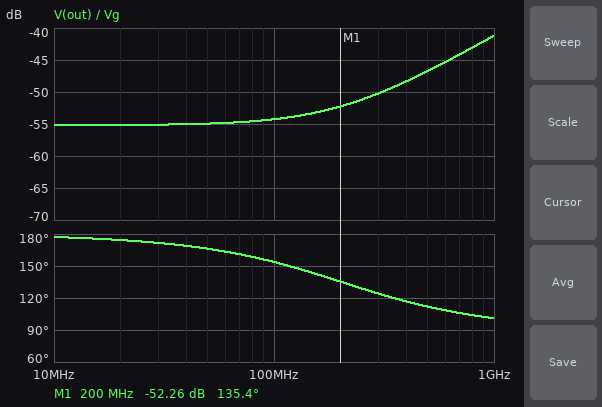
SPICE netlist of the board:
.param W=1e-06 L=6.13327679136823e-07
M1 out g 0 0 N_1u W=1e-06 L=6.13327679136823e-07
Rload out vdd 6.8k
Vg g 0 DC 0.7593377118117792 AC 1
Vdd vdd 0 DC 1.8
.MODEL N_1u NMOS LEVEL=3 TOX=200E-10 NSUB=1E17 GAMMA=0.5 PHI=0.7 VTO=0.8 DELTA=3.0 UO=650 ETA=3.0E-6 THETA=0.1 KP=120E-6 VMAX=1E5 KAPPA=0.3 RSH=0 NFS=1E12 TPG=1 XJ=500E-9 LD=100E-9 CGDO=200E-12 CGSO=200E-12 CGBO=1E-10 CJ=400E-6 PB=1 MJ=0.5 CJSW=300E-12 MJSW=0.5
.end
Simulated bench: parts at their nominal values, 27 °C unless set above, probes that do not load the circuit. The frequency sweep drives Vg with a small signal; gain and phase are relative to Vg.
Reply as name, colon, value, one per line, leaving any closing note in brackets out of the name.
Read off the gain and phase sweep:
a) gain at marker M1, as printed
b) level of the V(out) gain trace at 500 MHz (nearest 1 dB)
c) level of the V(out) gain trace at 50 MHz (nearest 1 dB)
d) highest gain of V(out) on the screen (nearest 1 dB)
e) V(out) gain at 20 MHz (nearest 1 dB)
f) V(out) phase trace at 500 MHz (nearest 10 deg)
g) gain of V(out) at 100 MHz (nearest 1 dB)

gain at marker M1, as printed: -52.26 dB
level of the V(out) gain trace at 500 MHz: -47 dB
level of the V(out) gain trace at 50 MHz: -55 dB
highest gain of V(out) on the screen: -41 dB
V(out) gain at 20 MHz: -55 dB
V(out) phase trace at 500 MHz: 110 deg
gain of V(out) at 100 MHz: -54 dB
